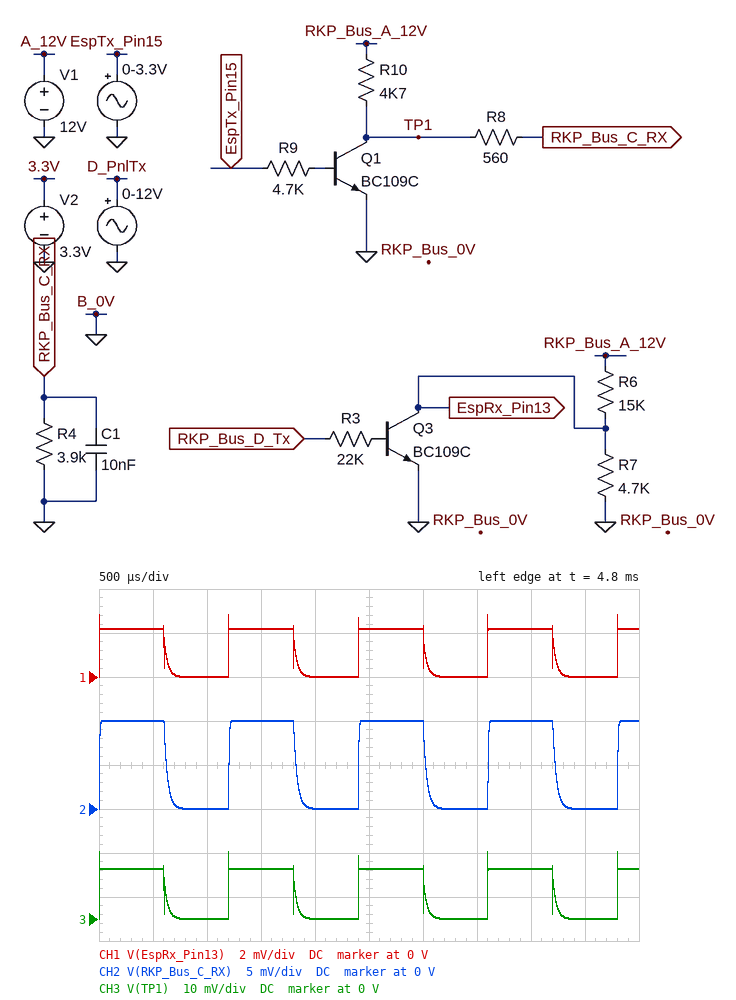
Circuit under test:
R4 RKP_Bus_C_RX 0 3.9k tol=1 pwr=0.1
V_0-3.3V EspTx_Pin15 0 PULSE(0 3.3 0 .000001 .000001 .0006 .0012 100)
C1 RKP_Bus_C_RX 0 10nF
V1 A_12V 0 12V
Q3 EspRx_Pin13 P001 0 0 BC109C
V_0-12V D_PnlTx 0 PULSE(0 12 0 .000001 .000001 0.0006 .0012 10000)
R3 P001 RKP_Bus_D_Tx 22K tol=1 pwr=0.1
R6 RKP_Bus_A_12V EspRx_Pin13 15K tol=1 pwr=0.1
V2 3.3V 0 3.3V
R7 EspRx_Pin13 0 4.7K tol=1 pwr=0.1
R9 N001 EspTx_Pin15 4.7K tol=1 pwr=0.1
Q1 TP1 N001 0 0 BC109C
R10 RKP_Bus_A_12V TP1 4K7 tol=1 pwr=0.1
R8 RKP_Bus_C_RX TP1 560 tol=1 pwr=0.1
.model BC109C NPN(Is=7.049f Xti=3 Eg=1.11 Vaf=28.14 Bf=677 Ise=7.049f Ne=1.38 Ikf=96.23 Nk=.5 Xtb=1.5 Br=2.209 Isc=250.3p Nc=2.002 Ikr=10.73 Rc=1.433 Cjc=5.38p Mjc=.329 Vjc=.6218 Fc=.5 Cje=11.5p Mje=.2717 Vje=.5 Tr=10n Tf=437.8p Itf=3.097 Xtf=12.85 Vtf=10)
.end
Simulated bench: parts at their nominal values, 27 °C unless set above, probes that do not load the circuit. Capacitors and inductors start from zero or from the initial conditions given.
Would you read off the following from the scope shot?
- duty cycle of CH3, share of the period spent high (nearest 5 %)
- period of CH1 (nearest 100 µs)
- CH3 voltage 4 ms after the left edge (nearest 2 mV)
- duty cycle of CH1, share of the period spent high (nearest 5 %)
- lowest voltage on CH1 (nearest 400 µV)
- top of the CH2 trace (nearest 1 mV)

50 %
1.2 ms
12 mV
50 %
0 V
10 mV
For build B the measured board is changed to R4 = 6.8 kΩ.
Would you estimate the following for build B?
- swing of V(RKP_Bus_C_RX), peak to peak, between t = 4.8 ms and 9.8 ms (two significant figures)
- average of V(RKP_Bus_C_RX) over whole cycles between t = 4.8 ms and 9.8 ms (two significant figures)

11 mV
5.7 mV
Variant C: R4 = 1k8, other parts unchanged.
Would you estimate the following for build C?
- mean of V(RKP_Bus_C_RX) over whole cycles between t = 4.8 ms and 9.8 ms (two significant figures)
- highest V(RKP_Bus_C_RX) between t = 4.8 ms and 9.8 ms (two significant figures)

4.4 mV
8.7 mV
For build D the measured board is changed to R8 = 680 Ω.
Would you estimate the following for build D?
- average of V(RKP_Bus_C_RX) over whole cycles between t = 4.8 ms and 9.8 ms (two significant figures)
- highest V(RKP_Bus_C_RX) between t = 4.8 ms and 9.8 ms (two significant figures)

5.1 mV
9.7 mV
